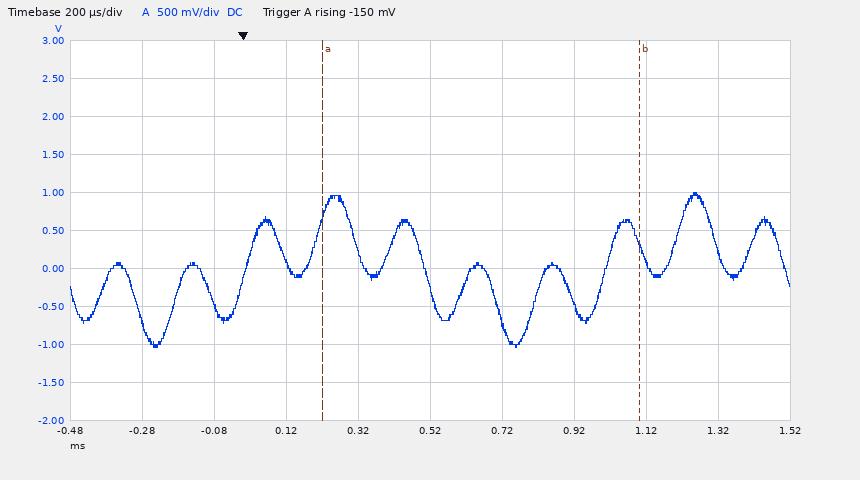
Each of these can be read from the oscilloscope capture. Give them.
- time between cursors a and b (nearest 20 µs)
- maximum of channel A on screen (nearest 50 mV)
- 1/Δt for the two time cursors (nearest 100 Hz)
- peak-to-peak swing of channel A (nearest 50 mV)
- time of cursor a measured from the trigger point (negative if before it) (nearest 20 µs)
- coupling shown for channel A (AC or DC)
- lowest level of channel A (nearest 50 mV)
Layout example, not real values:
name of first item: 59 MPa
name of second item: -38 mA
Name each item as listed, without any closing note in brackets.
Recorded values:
time between cursors a and b: 880 µs
maximum of channel A on screen: 1.00 V
1/Δt for the two time cursors: 1.1 kHz
peak-to-peak swing of channel A: 2.05 V
time of cursor a measured from the trigger point (negative if before it): +220 µs
coupling shown for channel A: DC
lowest level of channel A: -1.05 V
